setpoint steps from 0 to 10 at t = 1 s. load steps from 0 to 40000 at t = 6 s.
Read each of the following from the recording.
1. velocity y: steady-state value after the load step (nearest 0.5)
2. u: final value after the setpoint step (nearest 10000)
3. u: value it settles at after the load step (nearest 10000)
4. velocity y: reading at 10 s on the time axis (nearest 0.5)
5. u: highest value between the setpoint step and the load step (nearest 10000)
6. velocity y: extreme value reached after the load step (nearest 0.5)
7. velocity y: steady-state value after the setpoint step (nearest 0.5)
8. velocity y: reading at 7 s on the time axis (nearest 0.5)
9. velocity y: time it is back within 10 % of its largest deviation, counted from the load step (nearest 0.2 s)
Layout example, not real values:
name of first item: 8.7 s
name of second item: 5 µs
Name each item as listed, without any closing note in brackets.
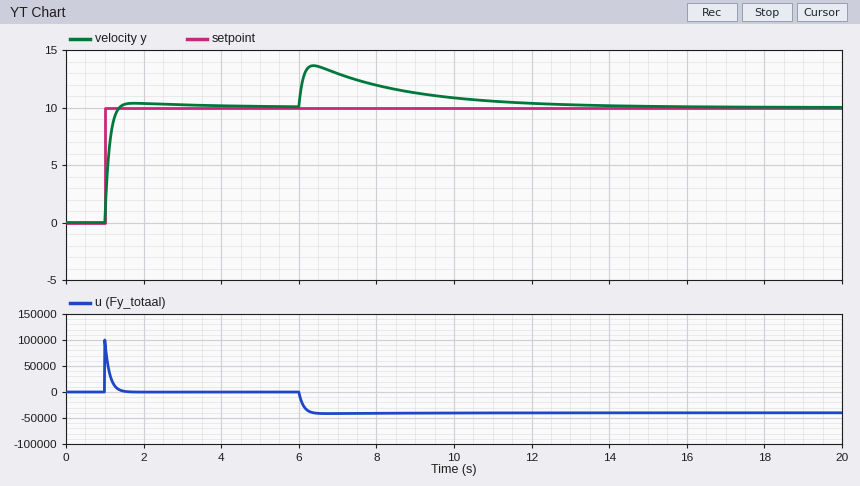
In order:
velocity y: steady-state value after the load step: 10.0
u: final value after the setpoint step: 0
u: value it settles at after the load step: -40000
velocity y: reading at 10 s on the time axis: 11.0
u: highest value between the setpoint step and the load step: 100000
velocity y: extreme value reached after the load step: 13.5
velocity y: steady-state value after the setpoint step: 10.0
velocity y: reading at 7 s on the time axis: 13.0
velocity y: time it is back within 10 % of its largest deviation, counted from the load step: 6.0 s
